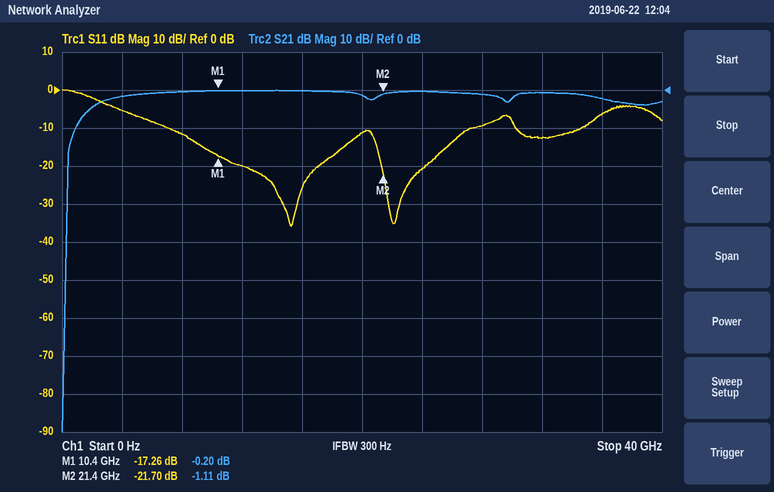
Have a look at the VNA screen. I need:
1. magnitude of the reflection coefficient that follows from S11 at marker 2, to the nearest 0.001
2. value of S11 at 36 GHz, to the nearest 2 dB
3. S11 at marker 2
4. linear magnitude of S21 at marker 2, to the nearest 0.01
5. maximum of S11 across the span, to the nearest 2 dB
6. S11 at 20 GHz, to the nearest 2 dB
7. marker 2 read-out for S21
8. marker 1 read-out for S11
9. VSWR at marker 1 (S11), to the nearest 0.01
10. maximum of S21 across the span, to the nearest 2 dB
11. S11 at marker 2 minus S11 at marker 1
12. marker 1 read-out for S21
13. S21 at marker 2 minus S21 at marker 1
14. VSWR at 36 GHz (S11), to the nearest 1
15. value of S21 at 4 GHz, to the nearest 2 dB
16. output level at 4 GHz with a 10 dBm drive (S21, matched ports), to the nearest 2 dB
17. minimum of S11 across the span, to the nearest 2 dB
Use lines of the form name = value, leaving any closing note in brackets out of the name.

magnitude of the reflection coefficient that follows from S11 at marker 2, to the nearest 0.001 = 0.082
value of S11 at 36 GHz, to the nearest 2 dB = -6 dB
S11 at marker 2 = -21.70 dB
linear magnitude of S21 at marker 2, to the nearest 0.01 = 0.88
maximum of S11 across the span, to the nearest 2 dB = 0 dB
S11 at 20 GHz, to the nearest 2 dB = -12 dB
marker 2 read-out for S21 = -1.11 dB
marker 1 read-out for S11 = -17.26 dB
VSWR at marker 1 (S11), to the nearest 0.01 = 1.32
maximum of S21 across the span, to the nearest 2 dB = 0 dB
S11 at marker 2 minus S11 at marker 1 = -4.44 dB
marker 1 read-out for S21 = -0.20 dB
S21 at marker 2 minus S21 at marker 1 = -0.91 dB
VSWR at 36 GHz (S11), to the nearest 1 = 3
value of S21 at 4 GHz, to the nearest 2 dB = -2 dB
output level at 4 GHz with a 10 dBm drive (S21, matched ports), to the nearest 2 dB = 8 dBm
minimum of S11 across the span, to the nearest 2 dB = -36 dB
